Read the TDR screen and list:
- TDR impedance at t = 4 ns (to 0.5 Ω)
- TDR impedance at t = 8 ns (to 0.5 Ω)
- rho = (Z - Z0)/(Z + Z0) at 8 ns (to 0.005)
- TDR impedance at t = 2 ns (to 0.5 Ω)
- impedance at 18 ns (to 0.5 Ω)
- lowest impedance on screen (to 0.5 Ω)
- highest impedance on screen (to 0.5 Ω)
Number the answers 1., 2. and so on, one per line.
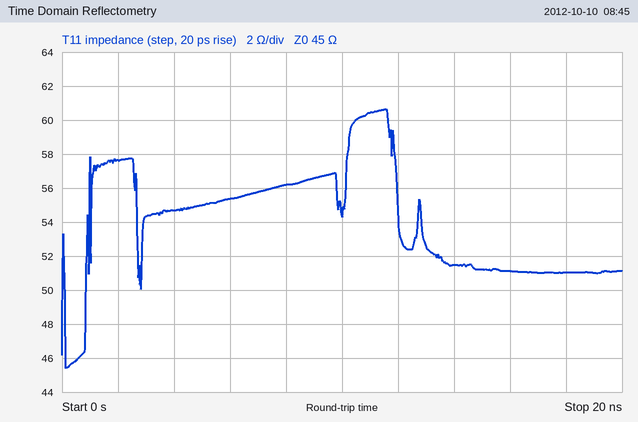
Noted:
1. 54.5 Ω
2. 56.0 Ω
3. +0.110
4. 57.5 Ω
5. 51.0 Ω
6. 45.5 Ω
7. 60.5 Ω
